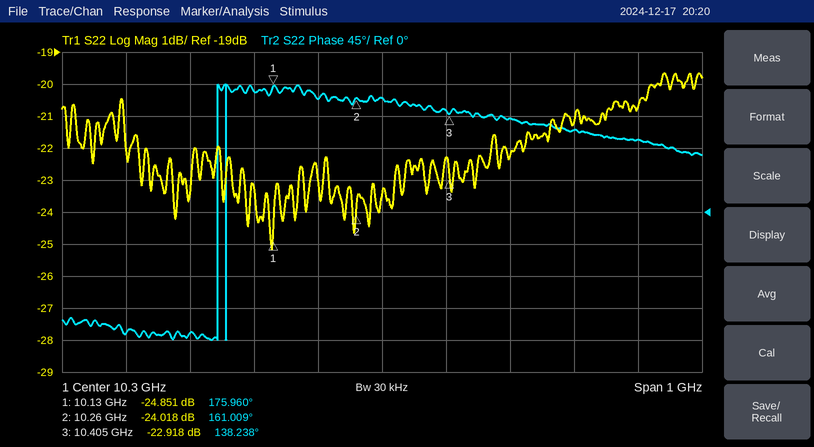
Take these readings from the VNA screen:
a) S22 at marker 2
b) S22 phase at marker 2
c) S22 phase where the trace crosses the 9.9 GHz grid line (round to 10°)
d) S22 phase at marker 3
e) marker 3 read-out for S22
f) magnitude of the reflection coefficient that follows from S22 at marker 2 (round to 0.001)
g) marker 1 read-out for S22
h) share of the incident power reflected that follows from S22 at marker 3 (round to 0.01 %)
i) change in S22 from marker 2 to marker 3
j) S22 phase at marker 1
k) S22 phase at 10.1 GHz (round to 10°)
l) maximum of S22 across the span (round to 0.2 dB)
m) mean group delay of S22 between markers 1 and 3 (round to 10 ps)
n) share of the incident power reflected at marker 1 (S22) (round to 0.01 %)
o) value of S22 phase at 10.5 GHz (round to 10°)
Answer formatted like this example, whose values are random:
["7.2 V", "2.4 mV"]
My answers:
["-24.018 dB", "161.009°", "-170°", "138.238°", "-22.918 dB", "0.063", "-24.851 dB", "0.51 %", "1.100 dB", "175.960°", "170°", "-19.6 dB", "380 ps", "0.33 %", "130°"]
